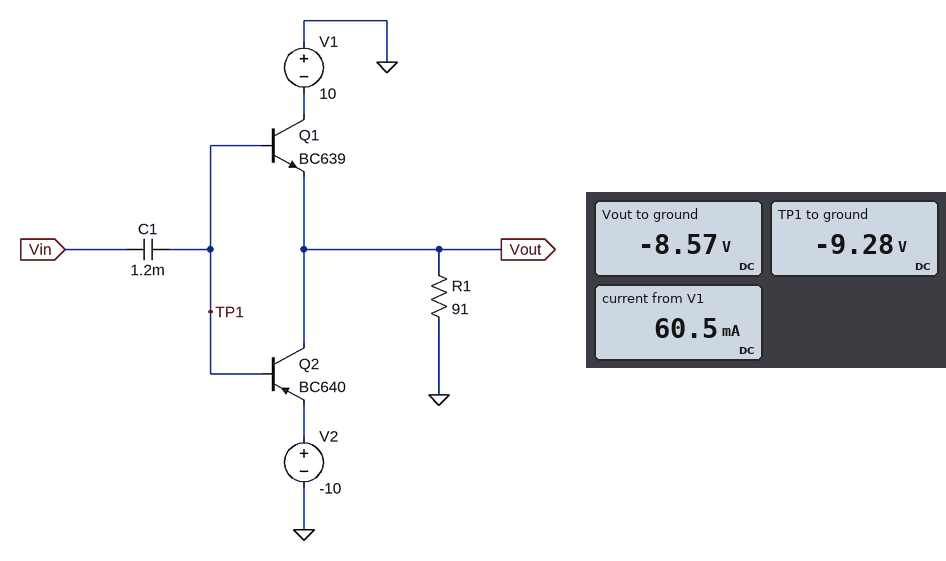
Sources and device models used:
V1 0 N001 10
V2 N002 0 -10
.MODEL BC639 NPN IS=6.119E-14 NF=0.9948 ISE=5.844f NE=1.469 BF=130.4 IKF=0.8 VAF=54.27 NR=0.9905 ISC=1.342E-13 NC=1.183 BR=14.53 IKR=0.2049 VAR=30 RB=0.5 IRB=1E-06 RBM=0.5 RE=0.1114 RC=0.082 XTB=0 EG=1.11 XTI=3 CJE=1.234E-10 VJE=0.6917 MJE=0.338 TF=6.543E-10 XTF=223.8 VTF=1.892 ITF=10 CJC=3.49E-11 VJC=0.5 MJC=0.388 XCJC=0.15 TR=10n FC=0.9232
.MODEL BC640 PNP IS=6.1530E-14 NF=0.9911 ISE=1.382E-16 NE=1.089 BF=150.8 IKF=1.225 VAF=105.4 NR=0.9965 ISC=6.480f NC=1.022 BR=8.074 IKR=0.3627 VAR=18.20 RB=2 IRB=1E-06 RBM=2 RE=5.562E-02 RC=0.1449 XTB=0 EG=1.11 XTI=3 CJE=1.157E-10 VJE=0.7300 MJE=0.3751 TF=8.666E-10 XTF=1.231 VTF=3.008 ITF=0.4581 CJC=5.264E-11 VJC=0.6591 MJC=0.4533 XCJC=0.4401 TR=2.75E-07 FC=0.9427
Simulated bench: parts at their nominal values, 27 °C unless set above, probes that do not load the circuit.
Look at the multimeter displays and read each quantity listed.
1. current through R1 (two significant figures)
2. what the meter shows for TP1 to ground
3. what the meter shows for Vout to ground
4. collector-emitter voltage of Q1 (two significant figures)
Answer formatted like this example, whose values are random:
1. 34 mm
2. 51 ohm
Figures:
1. 94 mA
2. -9.28 V
3. -8.57 V
4. -1.4 V
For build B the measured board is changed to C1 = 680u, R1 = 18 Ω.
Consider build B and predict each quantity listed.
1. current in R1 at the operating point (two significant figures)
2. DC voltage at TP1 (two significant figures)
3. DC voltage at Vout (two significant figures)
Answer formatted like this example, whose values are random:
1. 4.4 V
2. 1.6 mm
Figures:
1. 460 mA
2. -9.2 V
3. -8.3 V
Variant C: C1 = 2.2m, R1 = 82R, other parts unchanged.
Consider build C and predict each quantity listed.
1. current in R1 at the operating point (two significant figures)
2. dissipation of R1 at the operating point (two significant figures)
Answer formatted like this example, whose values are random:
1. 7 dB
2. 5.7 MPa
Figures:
1. 100 mA
2. 890 mW
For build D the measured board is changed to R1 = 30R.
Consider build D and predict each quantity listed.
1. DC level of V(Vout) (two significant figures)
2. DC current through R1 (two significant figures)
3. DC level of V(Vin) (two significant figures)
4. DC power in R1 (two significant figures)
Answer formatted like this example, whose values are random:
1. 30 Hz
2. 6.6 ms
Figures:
1. -8.4 V
2. 280 mA
3. -9.2 V
4. 2.4 W
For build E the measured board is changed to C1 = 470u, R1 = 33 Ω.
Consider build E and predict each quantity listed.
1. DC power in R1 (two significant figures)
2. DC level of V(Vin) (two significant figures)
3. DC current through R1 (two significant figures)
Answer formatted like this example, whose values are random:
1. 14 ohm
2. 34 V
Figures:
1. 2.2 W
2. -9.2 V
3. 260 mA
